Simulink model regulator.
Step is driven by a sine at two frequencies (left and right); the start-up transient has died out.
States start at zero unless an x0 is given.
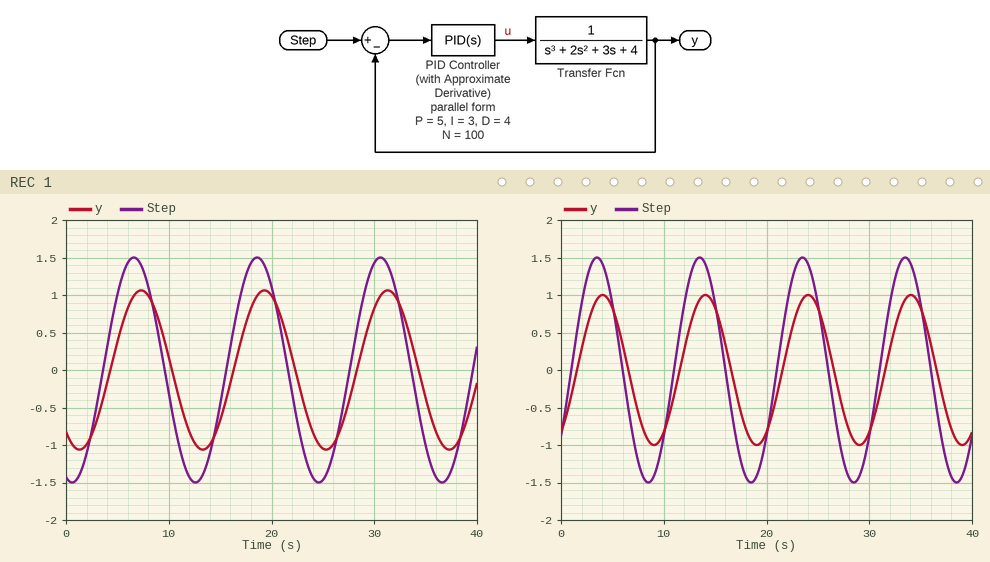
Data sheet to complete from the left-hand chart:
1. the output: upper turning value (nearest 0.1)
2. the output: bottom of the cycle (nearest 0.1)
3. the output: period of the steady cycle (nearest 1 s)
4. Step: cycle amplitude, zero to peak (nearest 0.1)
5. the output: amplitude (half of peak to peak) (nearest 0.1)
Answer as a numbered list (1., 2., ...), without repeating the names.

1. 1.1
2. -1.1
3. 12 s
4. 1.5
5. 1.1
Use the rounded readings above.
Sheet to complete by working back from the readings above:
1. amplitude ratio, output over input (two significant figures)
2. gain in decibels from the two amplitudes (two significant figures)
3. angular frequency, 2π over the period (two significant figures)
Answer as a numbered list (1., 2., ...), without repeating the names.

1. 0.73
2. -2.7 dB
3. 0.52 rad/s
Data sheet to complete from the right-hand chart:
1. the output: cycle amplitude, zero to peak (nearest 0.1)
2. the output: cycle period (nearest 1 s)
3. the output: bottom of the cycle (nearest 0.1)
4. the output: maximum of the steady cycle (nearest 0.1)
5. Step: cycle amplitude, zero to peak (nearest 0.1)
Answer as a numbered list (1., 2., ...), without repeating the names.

1. 1.0
2. 10 s
3. -1.0
4. 1.0
5. 1.5
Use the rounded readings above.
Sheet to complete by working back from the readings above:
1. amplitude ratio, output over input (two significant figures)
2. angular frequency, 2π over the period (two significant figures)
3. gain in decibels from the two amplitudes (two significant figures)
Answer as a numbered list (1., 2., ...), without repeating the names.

1. 0.67
2. 0.63 rad/s
3. -3.5 dB
